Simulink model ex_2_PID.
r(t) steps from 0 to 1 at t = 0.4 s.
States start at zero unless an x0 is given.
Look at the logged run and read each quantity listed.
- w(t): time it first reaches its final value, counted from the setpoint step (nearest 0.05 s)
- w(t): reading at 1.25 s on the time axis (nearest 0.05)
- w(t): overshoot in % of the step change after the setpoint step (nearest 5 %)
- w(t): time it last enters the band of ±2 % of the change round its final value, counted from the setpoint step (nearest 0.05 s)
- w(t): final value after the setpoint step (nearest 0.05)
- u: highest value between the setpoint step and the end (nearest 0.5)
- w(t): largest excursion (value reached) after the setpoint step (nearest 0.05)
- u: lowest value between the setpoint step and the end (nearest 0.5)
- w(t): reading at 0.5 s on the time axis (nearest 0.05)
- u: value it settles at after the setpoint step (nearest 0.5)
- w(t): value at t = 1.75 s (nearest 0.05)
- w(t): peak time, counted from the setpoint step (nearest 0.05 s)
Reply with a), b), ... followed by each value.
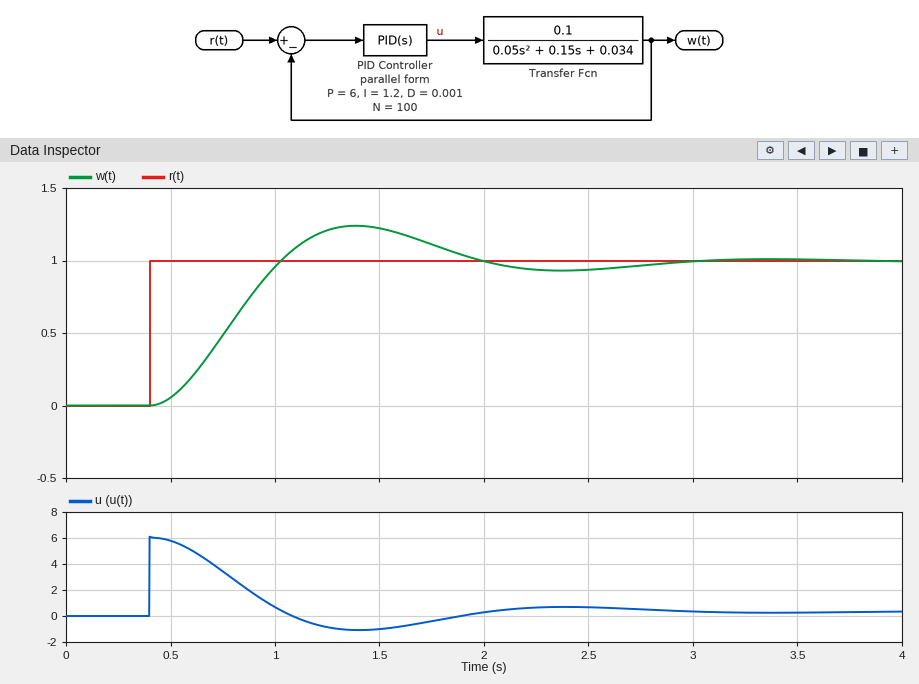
a) 0.65 s
b) 1.20
c) 25 %
d) 2.45 s
e) 1.00
f) 6.0
g) 1.25
h) -1.0
i) 0.05
j) 0.5
k) 1.10
l) 1.00 s
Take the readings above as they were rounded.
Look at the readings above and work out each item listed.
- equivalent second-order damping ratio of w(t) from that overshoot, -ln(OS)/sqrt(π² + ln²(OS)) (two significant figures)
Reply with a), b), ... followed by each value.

a) 0.40
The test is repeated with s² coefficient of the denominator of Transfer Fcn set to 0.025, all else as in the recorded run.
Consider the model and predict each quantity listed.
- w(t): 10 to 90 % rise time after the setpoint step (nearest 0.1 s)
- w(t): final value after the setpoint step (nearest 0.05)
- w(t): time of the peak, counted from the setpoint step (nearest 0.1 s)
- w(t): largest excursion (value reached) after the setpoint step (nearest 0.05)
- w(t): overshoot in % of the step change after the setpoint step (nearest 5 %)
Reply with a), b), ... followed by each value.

a) 0.4 s
b) 1.00
c) 0.8 s
d) 1.10
e) 10 %
